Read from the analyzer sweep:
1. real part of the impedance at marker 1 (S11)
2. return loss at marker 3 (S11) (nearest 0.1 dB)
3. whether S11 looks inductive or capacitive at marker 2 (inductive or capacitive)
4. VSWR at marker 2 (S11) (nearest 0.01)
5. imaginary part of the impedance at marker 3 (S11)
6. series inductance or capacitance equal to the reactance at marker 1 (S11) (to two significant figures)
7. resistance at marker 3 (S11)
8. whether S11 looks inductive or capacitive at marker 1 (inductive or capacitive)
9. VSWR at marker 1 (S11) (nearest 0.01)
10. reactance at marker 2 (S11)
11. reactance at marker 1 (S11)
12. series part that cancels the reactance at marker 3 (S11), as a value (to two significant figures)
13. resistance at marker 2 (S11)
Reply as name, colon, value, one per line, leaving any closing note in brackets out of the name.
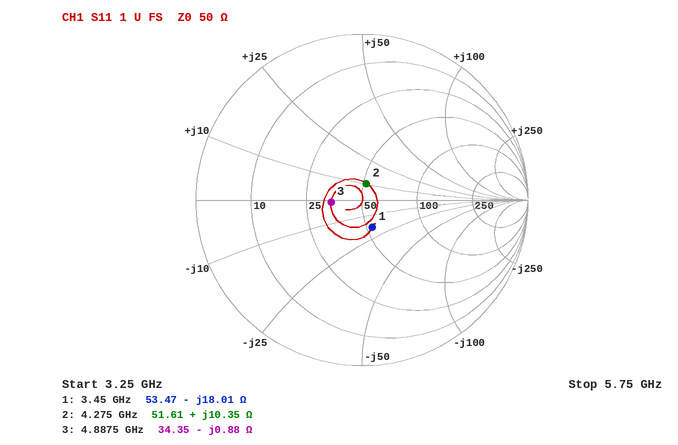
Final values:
real part of the impedance at marker 1: 53.47 Ω
return loss at marker 3 (S11): 14.6 dB
whether S11 looks inductive or capacitive at marker 2: inductive
VSWR at marker 2 (S11): 1.23
imaginary part of the impedance at marker 3: -0.88 Ω
series inductance or capacitance equal to the reactance at marker 1 (S11): 2.6 pF
resistance at marker 3: 34.35 Ω
whether S11 looks inductive or capacitive at marker 1: capacitive
VSWR at marker 1 (S11): 1.42
reactance at marker 2: +10.35 Ω
reactance at marker 1: -18.01 Ω
series part that cancels the reactance at marker 3 (S11), as a value: 29 pH
resistance at marker 2: 51.61 Ω
